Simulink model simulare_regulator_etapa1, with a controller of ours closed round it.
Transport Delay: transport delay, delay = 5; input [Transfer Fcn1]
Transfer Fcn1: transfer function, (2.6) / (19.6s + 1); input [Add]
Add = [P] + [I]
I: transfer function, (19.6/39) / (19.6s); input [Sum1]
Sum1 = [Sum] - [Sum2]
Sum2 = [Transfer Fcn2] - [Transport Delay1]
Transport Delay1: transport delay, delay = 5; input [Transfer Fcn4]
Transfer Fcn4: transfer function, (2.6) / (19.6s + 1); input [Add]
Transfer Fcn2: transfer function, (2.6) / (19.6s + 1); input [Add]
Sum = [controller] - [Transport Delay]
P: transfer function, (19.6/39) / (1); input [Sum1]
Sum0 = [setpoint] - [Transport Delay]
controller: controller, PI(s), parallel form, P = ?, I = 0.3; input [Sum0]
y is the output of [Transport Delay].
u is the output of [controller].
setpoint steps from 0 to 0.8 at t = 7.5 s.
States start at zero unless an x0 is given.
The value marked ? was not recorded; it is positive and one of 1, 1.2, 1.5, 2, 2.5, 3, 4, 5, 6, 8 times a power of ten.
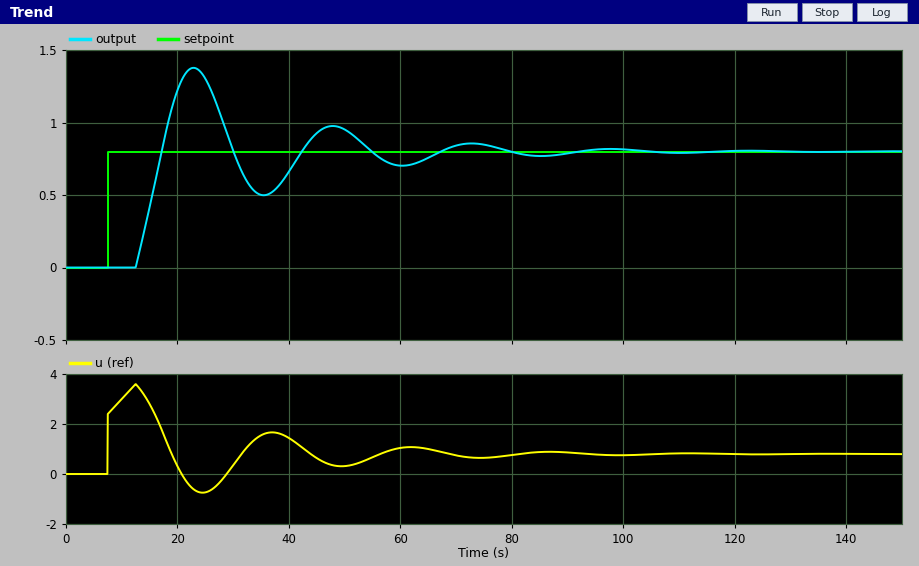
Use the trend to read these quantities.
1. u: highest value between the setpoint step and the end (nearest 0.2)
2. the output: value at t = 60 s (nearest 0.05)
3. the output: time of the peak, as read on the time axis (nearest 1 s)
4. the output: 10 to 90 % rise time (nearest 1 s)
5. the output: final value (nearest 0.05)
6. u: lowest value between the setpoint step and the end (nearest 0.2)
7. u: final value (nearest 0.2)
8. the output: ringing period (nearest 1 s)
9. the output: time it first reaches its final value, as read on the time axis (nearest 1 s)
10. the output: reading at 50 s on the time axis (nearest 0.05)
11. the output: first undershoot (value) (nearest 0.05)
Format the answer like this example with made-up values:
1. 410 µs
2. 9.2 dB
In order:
1. 3.6
2. 0.70
3. 23 s
4. 4 s
5. 0.80
6. -0.8
7. 0.8
8. 25 s
9. 17 s
10. 0.95
11. 0.50
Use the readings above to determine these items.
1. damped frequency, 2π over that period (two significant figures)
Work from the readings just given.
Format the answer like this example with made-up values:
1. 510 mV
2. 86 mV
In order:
1. 0.25 rad/s
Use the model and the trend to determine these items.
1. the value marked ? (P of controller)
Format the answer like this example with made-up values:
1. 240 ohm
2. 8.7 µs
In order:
1. 3
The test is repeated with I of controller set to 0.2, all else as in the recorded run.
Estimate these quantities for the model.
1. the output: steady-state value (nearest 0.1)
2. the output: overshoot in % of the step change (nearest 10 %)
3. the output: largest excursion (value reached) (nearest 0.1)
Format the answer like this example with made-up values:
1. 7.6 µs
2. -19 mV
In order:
1. 0.8
2. 50 %
3. 1.2
